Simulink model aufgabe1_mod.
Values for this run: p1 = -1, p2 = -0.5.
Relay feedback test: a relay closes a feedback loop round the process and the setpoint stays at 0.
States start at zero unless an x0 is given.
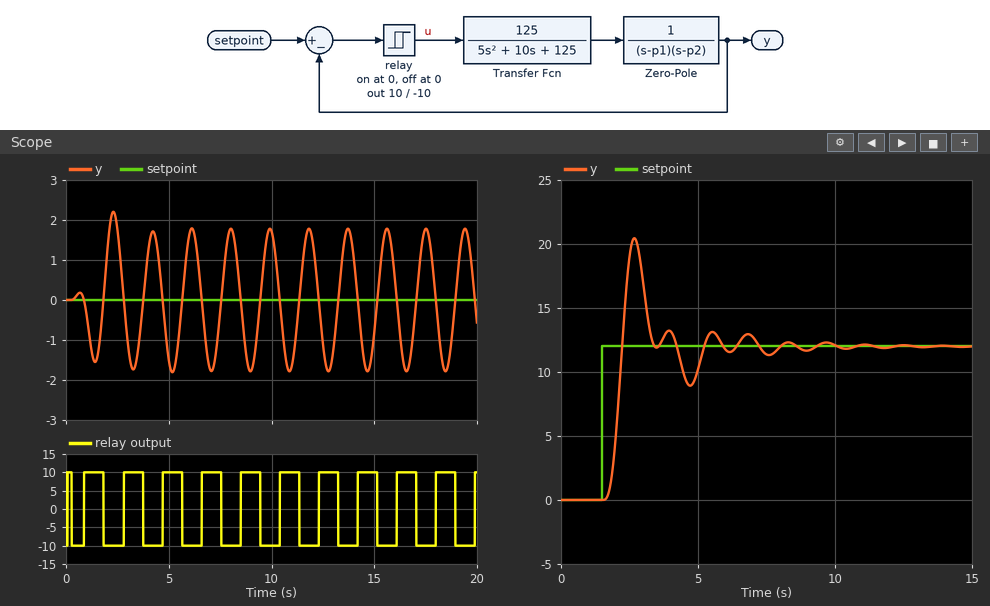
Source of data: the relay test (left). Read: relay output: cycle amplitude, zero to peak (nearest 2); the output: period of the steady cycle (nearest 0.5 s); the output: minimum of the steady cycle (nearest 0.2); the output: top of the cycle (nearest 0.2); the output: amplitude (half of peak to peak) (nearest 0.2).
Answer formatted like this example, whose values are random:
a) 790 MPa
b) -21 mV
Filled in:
a) 10
b) 2.0 s
c) -1.8
d) 1.8
e) 1.8
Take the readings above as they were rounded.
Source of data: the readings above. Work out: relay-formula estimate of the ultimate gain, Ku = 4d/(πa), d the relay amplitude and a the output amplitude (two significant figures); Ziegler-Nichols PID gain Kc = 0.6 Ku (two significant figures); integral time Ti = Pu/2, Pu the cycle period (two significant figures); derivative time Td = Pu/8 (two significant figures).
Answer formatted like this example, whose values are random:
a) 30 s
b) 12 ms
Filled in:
a) 7.1
b) 4.3
c) 1.0 s
d) 0.25 s
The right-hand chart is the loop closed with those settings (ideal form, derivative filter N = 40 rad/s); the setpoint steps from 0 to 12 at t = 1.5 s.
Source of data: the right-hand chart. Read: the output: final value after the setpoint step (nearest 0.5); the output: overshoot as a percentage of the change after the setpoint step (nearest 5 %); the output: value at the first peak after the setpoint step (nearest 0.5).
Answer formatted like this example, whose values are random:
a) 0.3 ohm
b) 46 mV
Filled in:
a) 12.0
b) 70 %
c) 20.5
